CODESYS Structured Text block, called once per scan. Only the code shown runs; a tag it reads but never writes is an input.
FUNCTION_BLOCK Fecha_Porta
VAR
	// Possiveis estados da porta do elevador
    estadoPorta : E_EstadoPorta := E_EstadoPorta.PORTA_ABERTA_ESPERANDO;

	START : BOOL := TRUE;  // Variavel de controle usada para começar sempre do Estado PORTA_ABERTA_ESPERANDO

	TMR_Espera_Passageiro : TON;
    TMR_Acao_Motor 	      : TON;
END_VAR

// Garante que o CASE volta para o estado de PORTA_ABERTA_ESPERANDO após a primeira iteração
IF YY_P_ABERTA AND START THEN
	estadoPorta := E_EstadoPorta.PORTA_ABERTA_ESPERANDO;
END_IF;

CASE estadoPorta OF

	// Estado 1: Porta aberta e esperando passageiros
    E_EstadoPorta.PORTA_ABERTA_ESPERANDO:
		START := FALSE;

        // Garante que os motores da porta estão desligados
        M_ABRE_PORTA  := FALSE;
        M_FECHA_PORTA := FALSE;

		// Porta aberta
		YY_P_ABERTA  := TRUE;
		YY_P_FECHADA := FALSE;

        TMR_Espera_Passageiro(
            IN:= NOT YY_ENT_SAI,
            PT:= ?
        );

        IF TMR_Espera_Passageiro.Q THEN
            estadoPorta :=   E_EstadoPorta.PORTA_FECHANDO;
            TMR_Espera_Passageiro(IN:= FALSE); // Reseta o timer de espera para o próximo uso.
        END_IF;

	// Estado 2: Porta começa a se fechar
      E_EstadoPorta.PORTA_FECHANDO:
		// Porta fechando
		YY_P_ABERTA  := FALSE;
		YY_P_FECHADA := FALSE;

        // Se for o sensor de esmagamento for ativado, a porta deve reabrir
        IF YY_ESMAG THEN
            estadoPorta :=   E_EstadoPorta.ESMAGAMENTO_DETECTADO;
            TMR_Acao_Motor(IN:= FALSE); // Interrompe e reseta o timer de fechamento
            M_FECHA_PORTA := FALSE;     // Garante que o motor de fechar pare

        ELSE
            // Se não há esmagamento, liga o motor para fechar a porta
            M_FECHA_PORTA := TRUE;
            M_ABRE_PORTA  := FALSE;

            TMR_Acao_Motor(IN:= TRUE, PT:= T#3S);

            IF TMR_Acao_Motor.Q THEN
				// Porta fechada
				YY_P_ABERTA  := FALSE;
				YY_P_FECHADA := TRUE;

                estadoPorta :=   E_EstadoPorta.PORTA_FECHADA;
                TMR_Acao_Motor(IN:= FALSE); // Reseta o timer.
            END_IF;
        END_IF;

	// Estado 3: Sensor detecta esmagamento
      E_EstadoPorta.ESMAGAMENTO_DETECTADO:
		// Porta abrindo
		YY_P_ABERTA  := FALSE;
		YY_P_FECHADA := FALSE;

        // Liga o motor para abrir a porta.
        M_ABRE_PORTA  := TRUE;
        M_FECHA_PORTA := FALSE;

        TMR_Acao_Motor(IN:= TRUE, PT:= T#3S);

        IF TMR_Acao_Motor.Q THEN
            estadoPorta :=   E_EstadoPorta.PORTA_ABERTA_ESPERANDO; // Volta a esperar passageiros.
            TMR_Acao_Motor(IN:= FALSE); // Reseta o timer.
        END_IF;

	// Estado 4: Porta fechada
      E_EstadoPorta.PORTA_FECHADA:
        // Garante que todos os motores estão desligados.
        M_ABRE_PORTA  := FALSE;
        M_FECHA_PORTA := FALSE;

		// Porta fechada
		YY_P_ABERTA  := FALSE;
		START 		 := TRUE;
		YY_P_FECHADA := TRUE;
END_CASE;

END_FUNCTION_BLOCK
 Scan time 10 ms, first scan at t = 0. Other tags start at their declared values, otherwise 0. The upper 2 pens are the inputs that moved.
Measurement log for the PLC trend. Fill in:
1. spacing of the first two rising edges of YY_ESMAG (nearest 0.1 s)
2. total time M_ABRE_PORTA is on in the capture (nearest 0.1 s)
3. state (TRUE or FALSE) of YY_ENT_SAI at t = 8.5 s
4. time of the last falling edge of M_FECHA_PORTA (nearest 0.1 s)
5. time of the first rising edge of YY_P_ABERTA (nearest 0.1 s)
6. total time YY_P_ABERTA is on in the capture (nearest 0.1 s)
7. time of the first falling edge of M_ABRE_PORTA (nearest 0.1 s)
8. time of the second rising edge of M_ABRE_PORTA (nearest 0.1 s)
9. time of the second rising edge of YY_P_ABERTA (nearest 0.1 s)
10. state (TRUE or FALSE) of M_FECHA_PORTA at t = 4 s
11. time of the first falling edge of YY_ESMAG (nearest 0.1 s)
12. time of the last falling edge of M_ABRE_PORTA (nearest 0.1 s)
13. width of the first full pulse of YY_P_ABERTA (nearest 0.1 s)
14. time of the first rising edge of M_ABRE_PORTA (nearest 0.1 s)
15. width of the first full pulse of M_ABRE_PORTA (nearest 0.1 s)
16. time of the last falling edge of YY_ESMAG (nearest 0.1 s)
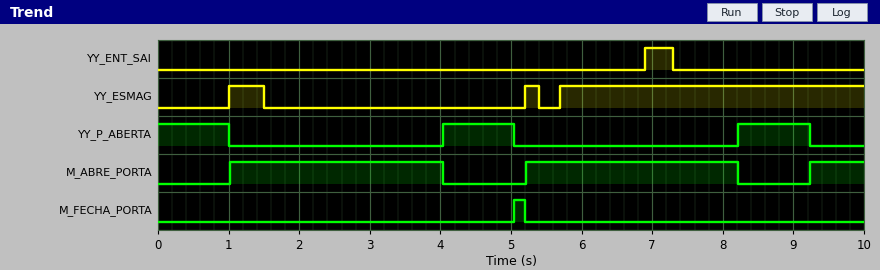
4.2 s
6.8 s
FALSE
5.2 s
4.0 s
3.0 s
4.0 s
5.2 s
8.2 s
FALSE
1.5 s
8.2 s
1.0 s
1.0 s
3.0 s
5.4 s
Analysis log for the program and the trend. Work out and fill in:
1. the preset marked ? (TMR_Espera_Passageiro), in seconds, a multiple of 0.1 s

1.0 s
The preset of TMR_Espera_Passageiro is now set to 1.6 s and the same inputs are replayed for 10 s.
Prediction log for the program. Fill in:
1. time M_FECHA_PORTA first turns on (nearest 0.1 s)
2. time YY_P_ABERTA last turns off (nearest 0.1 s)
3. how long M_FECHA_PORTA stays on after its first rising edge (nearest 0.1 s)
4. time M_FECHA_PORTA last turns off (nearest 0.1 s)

1.6 s
1.6 s
3.0 s
4.6 s
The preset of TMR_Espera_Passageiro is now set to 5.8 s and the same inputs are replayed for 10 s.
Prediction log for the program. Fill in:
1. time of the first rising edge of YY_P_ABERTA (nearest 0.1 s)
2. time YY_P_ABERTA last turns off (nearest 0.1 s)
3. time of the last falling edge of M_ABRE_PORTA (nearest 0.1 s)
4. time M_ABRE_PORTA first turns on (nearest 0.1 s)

8.8 s
5.8 s
8.8 s
5.8 s
